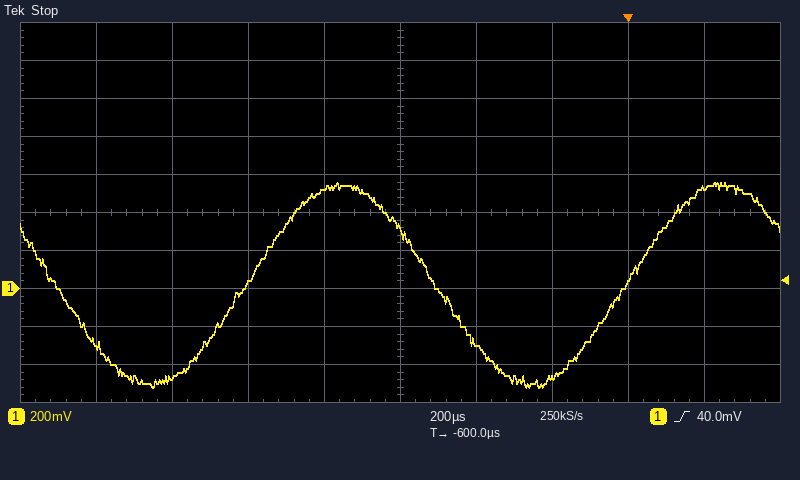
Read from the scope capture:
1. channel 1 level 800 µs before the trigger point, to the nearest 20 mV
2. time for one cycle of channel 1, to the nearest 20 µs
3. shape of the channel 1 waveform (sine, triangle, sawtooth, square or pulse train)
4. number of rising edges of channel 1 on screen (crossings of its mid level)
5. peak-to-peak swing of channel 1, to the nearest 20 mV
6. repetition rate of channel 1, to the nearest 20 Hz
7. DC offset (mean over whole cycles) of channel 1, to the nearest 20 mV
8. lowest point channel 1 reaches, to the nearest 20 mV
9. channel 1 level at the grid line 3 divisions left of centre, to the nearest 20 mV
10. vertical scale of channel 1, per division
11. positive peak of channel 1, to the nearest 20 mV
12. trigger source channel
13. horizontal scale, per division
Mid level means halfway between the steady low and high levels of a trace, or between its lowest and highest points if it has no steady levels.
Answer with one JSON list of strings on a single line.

["520 mV", "1.00 ms", "sine", "2", "1.08 V", "1.00 kHz", "20 mV", "-520 mV", "-480 mV", "200 mV", "560 mV", "channel 1", "200 µs"]
